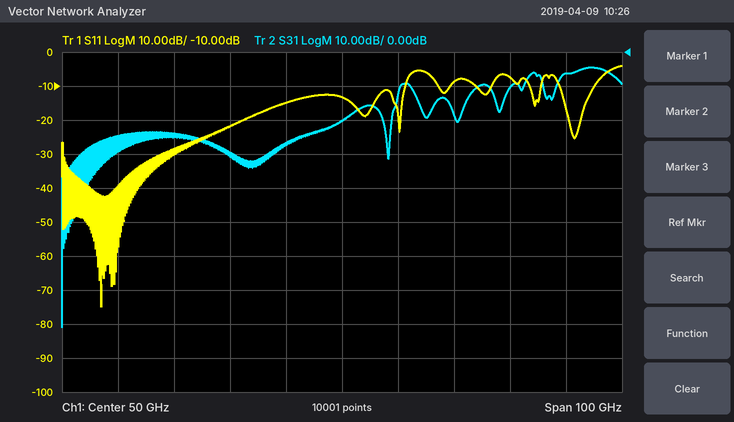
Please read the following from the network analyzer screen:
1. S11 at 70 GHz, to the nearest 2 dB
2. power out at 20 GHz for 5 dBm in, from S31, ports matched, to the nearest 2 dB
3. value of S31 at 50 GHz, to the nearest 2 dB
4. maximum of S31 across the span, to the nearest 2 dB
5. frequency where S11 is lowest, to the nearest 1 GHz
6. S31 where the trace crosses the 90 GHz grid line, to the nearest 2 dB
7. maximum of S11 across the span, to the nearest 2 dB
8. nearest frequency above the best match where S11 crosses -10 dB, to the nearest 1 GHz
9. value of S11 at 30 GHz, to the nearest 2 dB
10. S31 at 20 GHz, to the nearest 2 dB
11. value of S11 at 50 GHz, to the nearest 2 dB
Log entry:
-8 dB
-20 dBm
-20 dB
-4 dB
7 GHz
-6 dB
-4 dB
61 GHz
-22 dB
-24 dB
-14 dB
